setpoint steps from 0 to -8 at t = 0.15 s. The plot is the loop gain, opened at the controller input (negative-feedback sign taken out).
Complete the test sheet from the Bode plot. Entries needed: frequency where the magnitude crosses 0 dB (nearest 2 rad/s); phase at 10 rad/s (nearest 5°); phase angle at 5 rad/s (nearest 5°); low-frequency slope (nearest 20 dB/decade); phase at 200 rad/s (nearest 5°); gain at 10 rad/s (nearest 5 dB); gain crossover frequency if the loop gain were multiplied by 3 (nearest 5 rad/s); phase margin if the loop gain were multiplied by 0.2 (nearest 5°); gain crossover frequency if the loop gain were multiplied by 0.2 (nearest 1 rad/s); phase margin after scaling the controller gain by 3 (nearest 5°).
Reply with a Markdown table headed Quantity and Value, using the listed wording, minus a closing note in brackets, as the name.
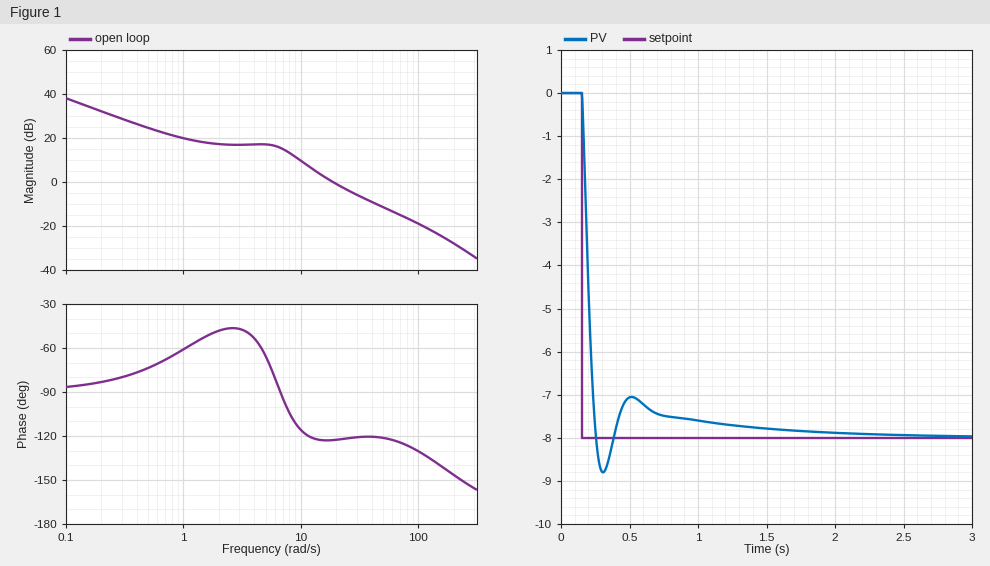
| Quantity | Value |
|---|---|
| frequency where the magnitude crosses 0 dB | 18 rad/s |
| phase at 10 rad/s | -115° |
| phase angle at 5 rad/s | -65° |
| low-frequency slope | -20 dB/decade |
| phase at 200 rad/s | -145° |
| gain at 10 rad/s | 10 dB |
| gain crossover frequency if the loop gain were multiplied by 3 | 40 rad/s |
| phase margin if the loop gain were multiplied by 0.2 | 80° |
| gain crossover frequency if the loop gain were multiplied by 0.2 | 8 rad/s |
| phase margin after scaling the controller gain by 3 | 60° |
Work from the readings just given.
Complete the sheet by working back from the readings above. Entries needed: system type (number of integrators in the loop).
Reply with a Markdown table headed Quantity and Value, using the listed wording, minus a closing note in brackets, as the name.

| Quantity | Value |
|---|---|
| system type | 1 |
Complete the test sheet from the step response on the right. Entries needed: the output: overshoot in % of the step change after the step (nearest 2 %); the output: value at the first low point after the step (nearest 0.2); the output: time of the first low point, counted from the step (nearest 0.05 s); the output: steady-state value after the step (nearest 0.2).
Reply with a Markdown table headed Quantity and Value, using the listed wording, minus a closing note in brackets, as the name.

| Quantity | Value |
|---|---|
| the output: overshoot in % of the step change after the step | 10 % |
| the output: value at the first low point after the step | -8.8 |
| the output: time of the first low point, counted from the step | 0.15 s |
| the output: steady-state value after the step | -8.0 |
